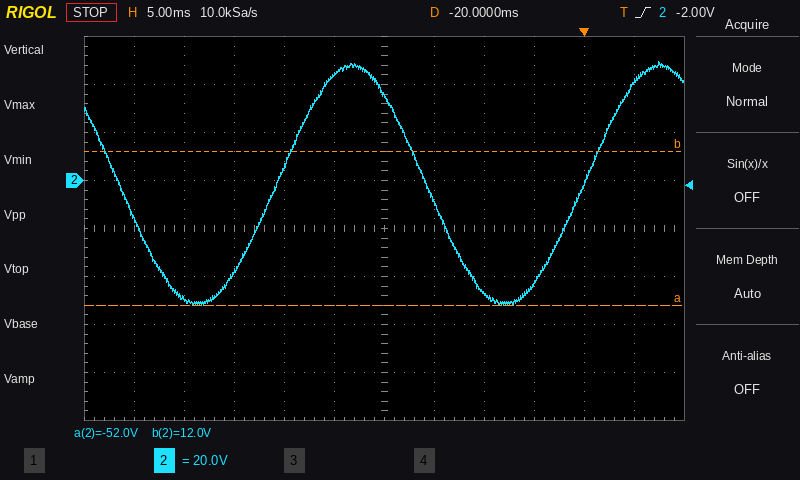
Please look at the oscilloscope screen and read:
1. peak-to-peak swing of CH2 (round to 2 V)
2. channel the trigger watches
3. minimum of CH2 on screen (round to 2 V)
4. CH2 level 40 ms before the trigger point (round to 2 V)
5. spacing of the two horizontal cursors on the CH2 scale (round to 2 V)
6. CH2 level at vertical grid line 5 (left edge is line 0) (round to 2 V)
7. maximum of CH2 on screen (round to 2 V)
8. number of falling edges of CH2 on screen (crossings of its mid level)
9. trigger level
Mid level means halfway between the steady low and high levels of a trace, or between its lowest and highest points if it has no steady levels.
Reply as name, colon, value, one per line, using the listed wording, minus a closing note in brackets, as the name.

peak-to-peak swing of CH2: 102 V
channel the trigger watches: CH2
minimum of CH2 on screen: -52 V
CH2 level 40 ms before the trigger point: -50 V
spacing of the two horizontal cursors on the CH2 scale: 64 V
CH2 level at vertical grid line 5 (left edge is line 0): 44 V
maximum of CH2 on screen: 50 V
number of falling edges of CH2 on screen: 2
trigger level: -2.00 V
